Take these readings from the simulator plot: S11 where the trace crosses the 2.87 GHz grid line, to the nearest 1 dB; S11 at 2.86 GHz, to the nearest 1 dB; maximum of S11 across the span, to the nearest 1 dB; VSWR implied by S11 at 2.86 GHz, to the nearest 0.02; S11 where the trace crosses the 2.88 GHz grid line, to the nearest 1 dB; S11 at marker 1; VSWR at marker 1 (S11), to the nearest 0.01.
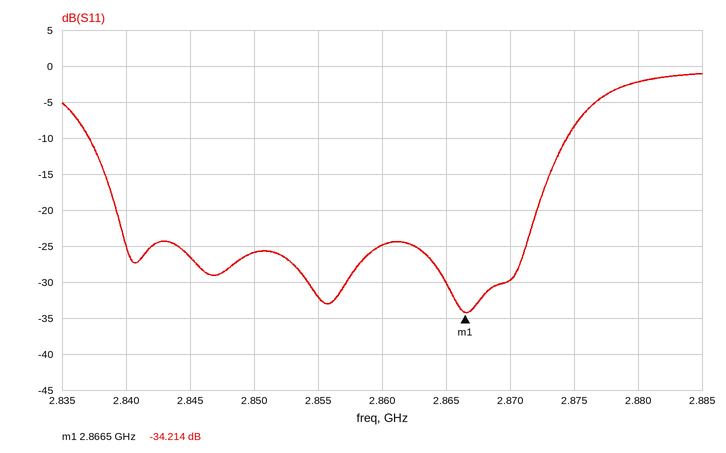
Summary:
-30 dB
-25 dB
-1 dB
1.12
-2 dB
-34.214 dB
1.04
